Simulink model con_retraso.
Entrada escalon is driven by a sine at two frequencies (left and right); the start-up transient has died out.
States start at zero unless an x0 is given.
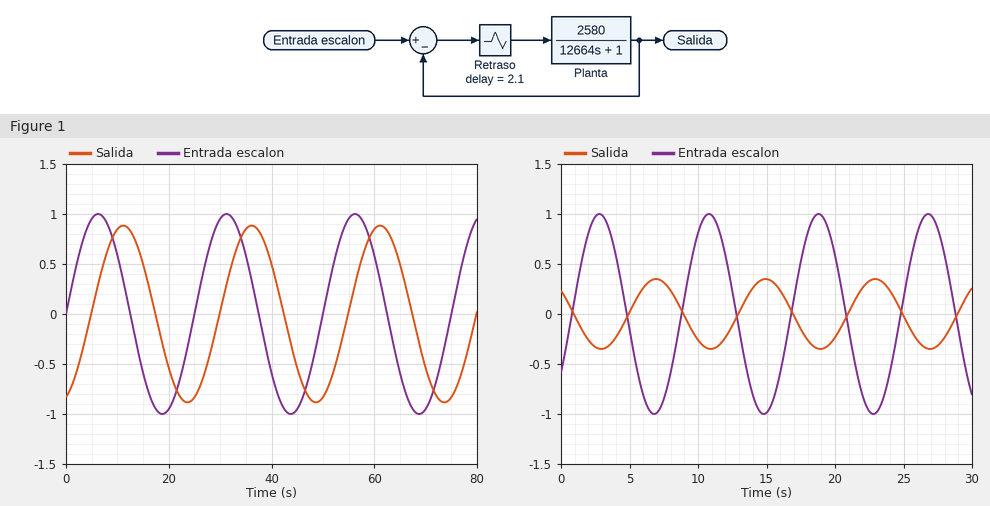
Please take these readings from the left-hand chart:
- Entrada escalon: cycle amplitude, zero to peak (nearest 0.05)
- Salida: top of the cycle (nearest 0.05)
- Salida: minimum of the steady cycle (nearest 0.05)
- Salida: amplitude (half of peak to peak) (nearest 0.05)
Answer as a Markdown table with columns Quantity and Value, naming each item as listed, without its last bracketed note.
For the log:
| Quantity | Value |
|---|---|
| Entrada escalon: cycle amplitude, zero to peak | 1.00 |
| Salida: top of the cycle | 0.90 |
| Salida: minimum of the steady cycle | -0.90 |
| Salida: amplitude (half of peak to peak) | 0.90 |
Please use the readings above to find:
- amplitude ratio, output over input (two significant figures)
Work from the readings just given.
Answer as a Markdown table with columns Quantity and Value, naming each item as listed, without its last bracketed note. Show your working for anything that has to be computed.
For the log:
| Quantity | Value |
|---|---|
| amplitude ratio, output over input | 0.9 / 1 = 0.90 |
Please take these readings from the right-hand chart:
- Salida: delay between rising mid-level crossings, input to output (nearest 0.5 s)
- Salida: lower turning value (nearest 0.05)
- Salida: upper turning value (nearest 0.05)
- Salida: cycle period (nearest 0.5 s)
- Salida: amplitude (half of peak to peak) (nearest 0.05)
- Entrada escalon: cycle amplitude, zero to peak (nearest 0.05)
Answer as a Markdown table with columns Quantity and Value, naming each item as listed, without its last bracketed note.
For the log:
| Quantity | Value |
|---|---|
| Salida: delay between rising mid-level crossings, input to output | 4.0 s |
| Salida: lower turning value | -0.35 |
| Salida: upper turning value | 0.35 |
| Salida: cycle period | 8.0 s |
| Salida: amplitude (half of peak to peak) | 0.35 |
| Entrada escalon: cycle amplitude, zero to peak | 1.00 |
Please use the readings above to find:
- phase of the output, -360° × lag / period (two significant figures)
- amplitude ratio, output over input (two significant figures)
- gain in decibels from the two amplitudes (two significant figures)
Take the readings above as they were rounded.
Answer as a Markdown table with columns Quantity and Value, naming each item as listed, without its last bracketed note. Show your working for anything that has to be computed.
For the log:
| Quantity | Value |
|---|---|
| phase of the output, -360° × lag / period | -360 × 4 / 8 = -180° |
| amplitude ratio, output over input | 0.35 / 1 = 0.35 |
| gain in decibels from the two amplitudes | 20 log10(0.35 / 1) = -9.1 dB |
